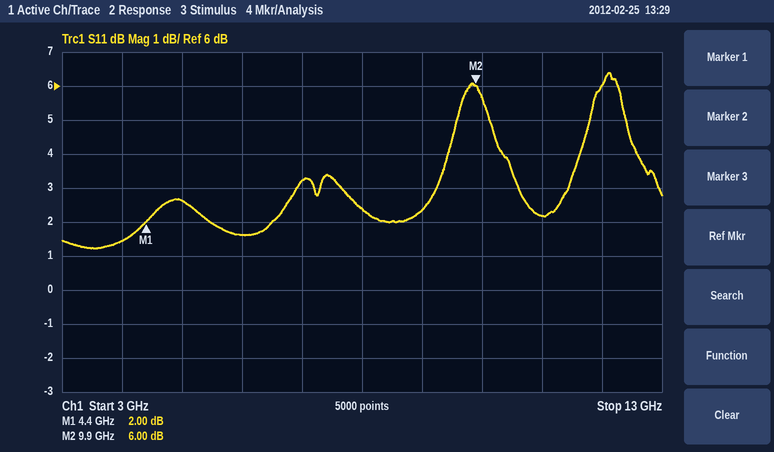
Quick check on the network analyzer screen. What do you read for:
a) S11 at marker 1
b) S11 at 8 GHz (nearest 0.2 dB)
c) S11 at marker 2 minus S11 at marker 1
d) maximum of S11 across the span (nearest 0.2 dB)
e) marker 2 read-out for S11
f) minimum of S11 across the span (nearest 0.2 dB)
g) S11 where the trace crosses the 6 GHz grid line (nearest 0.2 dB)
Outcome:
2.00 dB
2.4 dB
4.00 dB
6.4 dB
6.00 dB
1.2 dB
1.6 dB
